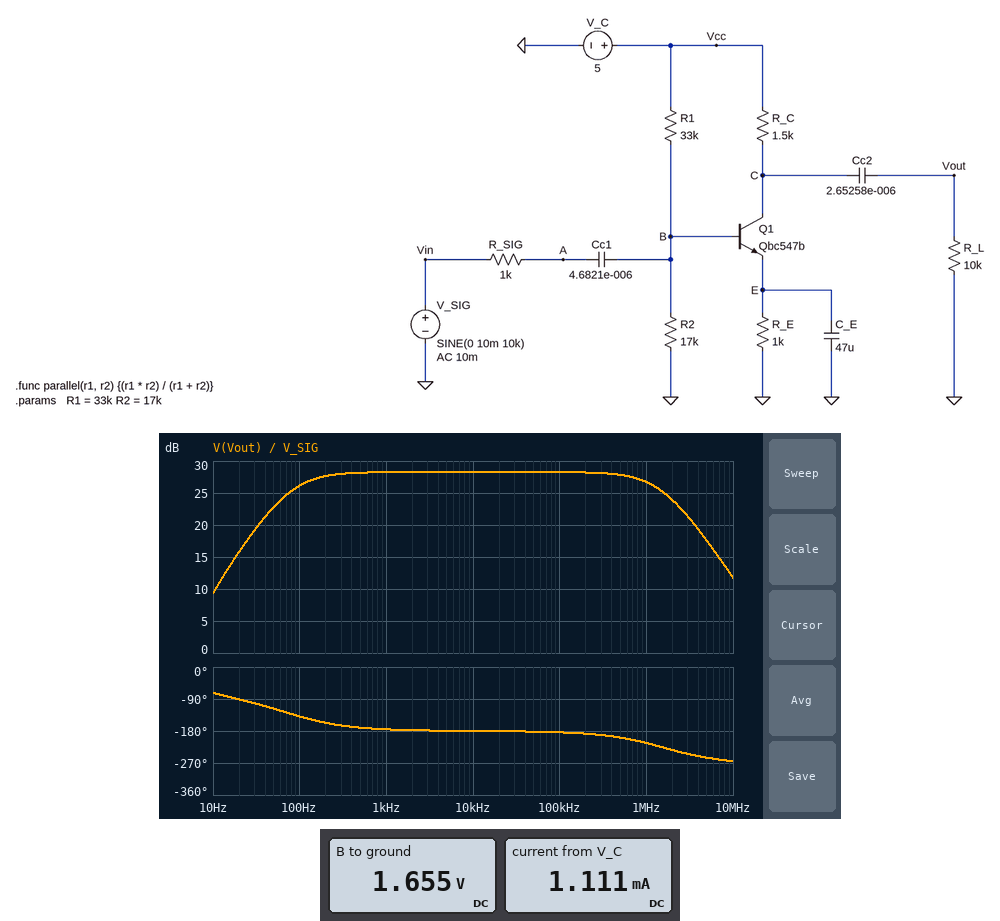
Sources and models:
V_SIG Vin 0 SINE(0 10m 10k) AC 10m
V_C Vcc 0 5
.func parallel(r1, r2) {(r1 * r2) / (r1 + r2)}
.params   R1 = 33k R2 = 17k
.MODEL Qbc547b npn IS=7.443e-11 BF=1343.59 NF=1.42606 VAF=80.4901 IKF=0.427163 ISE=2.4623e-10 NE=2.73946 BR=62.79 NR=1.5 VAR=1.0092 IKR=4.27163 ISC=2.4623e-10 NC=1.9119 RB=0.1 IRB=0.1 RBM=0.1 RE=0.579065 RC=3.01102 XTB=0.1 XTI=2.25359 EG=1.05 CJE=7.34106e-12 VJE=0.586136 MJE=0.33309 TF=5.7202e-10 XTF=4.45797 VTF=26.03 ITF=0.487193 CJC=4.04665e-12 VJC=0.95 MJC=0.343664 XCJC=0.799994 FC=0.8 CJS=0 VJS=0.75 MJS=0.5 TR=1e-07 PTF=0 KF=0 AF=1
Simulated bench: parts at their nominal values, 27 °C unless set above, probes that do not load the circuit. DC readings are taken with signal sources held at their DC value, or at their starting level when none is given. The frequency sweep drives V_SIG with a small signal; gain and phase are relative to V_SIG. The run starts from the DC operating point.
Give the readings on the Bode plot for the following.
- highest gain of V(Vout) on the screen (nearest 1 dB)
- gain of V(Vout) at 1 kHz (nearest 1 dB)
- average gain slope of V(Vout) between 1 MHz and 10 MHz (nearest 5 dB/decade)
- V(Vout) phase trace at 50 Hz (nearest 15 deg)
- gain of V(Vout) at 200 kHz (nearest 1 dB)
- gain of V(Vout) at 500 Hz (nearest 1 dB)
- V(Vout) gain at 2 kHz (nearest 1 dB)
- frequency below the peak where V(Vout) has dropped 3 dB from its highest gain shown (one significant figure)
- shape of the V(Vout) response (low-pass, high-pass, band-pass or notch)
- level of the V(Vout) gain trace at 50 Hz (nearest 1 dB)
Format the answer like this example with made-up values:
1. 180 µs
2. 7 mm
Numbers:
1. 28 dB
2. 28 dB
3. -15 dB/decade
4. -120 deg
5. 28 dB
6. 28 dB
7. 28 dB
8. 80 Hz
9. band-pass
10. 23 dB
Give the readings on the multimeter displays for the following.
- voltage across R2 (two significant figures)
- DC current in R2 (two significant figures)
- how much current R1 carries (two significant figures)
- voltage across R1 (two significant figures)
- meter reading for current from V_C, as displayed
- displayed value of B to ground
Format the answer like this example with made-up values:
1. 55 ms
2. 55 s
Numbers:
1. 1.7 V
2. 97 µA
3. 100 µA
4. 3.3 V
5. 1.111 mA
6. 1.655 V
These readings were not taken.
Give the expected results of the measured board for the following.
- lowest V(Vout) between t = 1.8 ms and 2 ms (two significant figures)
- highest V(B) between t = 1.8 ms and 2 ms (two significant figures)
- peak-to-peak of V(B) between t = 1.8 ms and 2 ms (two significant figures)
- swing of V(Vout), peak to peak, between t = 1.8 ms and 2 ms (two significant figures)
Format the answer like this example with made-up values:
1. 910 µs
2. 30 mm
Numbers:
1. -270 mV
2. 1.7 V
3. 17 mV
4. 520 mV
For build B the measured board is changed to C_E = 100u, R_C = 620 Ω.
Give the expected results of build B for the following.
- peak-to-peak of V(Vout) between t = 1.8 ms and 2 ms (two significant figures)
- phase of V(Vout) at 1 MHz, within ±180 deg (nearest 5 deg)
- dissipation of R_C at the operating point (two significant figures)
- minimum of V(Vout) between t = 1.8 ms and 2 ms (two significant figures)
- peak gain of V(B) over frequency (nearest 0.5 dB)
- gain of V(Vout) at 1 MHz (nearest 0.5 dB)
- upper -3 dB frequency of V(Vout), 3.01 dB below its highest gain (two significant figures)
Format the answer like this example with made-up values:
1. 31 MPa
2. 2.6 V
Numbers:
1. 240 mV
2. 160 deg
3. 630 µW
4. -130 mV
5. -1.5 dB
6. 21.0 dB
7. 2.6 MHz
